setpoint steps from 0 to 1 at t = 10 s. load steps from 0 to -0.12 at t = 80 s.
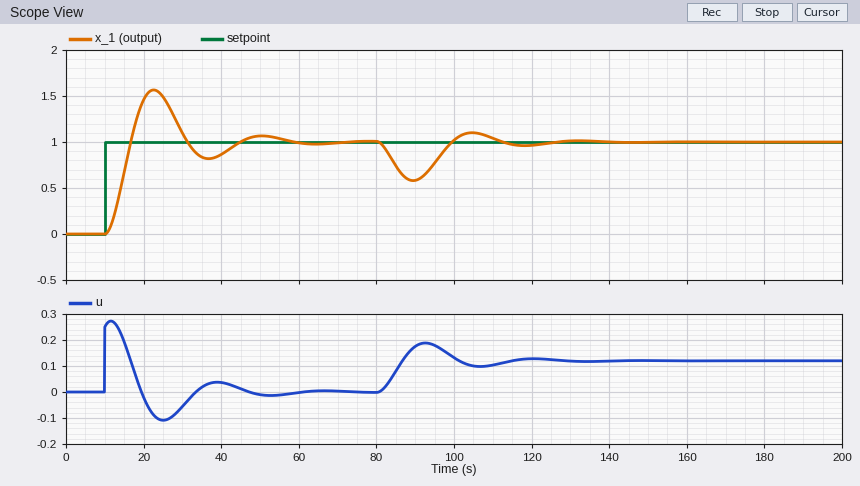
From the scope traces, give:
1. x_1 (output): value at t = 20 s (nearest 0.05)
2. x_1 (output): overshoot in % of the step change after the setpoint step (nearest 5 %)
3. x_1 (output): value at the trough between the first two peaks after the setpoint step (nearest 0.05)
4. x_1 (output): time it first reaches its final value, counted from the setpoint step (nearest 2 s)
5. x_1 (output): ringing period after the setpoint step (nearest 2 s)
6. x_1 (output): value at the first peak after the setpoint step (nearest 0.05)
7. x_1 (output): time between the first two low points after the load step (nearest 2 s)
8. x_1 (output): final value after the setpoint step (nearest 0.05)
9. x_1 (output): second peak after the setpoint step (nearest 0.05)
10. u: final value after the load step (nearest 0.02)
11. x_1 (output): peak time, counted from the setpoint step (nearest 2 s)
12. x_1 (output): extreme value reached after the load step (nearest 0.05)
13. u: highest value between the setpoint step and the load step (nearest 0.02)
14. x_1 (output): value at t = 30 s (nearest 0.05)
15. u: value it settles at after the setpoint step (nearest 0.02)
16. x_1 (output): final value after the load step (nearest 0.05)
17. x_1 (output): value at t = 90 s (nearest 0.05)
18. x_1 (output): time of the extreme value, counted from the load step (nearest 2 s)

1.45
55 %
0.80
6 s
28 s
1.55
28 s
1.00
1.05
0.12
12 s
0.60
0.28
1.10
0.00
1.00
0.60
10 s
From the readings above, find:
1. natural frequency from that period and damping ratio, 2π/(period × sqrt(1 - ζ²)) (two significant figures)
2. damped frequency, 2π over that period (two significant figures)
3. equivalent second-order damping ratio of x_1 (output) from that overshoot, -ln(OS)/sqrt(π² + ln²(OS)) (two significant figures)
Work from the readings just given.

0.23 rad/s
0.22 rad/s
0.19
